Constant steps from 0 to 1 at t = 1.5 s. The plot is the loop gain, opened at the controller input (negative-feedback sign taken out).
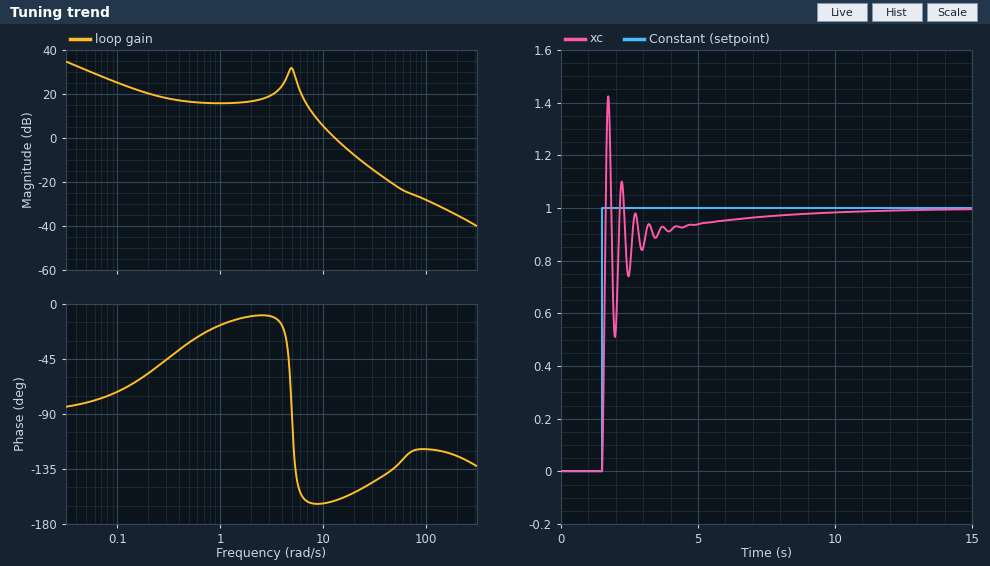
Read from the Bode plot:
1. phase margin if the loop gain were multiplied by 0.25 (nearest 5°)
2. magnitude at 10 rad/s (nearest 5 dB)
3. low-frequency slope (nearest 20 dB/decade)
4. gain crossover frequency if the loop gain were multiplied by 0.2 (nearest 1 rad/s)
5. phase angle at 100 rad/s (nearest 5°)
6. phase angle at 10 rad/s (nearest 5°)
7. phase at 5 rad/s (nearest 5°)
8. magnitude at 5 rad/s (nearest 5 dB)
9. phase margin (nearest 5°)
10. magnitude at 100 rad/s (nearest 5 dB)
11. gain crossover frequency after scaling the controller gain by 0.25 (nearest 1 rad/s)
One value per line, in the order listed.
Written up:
15°
5 dB
-20 dB/decade
7 rad/s
-120°
-165°
-90°
30 dB
20°
-30 dB
8 rad/s
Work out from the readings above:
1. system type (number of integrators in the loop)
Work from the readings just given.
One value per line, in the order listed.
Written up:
1
